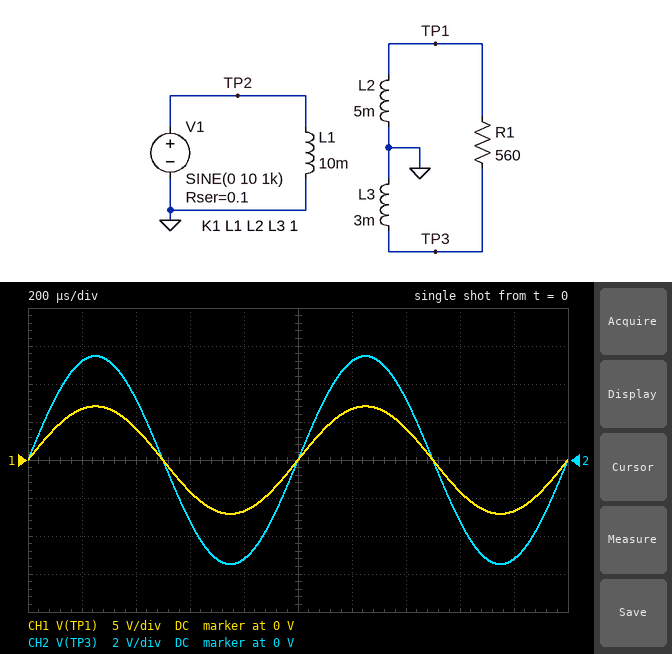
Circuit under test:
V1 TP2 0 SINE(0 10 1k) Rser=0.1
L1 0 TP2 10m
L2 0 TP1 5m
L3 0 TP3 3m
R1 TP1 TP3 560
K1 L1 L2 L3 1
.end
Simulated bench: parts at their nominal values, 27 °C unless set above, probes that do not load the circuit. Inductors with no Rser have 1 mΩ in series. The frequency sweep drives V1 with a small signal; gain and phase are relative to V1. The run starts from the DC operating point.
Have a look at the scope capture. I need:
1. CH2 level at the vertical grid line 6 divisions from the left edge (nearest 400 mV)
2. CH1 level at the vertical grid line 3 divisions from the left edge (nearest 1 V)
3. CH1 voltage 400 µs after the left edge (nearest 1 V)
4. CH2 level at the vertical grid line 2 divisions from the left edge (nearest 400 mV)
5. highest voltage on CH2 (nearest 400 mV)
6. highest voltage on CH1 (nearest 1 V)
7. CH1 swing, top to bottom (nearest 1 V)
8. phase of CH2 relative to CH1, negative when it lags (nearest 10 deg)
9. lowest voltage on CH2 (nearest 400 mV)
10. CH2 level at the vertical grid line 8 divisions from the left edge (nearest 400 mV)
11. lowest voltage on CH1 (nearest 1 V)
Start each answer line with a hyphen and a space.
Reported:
- 5.2 V
- -4 V
- 4 V
- 3.2 V
- 5.6 V
- 7 V
- 14 V
- 0 deg
- -5.6 V
- -3.2 V
- -7 V
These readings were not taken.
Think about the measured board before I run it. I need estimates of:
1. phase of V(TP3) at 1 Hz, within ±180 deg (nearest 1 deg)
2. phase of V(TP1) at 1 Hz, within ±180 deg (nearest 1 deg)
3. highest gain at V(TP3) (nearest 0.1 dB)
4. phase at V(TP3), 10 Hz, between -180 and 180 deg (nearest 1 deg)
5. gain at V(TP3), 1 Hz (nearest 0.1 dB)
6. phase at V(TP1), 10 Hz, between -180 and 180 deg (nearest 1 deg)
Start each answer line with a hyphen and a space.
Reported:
- 58 deg
- 58 deg
- -5.2 dB
- 9 deg
- -10.8 dB
- 9 deg
